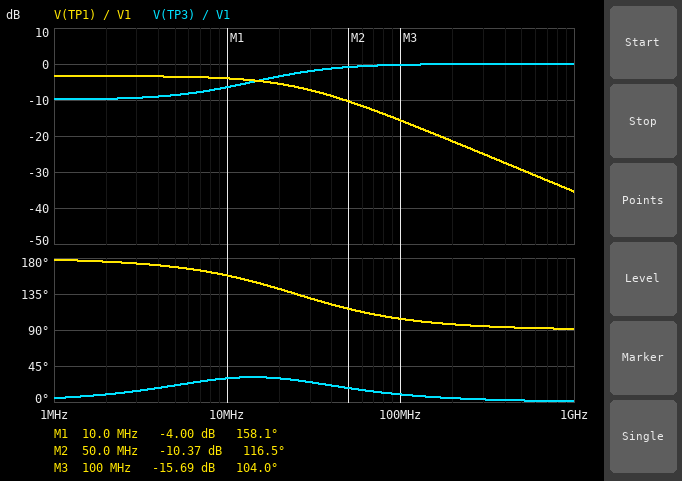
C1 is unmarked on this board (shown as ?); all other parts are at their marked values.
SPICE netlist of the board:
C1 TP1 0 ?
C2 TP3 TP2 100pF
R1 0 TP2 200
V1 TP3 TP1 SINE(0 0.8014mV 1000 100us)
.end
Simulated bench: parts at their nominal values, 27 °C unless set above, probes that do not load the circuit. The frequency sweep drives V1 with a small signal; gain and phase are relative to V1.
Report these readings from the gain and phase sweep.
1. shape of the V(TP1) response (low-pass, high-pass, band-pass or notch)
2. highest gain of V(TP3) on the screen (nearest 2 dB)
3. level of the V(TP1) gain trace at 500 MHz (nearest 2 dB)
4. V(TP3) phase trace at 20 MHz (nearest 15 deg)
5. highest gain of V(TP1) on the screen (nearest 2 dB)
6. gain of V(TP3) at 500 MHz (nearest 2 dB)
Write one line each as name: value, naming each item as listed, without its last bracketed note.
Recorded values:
shape of the V(TP1) response: low-pass
highest gain of V(TP3) on the screen: 0 dB
level of the V(TP1) gain trace at 500 MHz: -30 dB
V(TP3) phase trace at 20 MHz: 30 deg
highest gain of V(TP1) on the screen: -4 dB
gain of V(TP3) at 500 MHz: 0 dB
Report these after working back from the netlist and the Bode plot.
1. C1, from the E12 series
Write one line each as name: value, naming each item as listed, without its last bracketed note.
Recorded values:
C1, from the E12 series: 47 pF
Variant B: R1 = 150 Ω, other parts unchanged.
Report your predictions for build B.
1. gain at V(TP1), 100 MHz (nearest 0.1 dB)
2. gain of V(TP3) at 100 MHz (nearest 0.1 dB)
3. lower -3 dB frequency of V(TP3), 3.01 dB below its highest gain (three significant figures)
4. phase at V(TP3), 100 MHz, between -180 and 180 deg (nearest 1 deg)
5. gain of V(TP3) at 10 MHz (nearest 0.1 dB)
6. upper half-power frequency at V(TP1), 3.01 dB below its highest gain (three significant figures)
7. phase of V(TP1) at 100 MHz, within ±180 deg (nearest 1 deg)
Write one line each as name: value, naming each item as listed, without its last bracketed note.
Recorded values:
gain at V(TP1), 100 MHz: -13.4 dB
gain of V(TP3) at 100 MHz: -0.4 dB
lower -3 dB frequency of V(TP3), 3.01 dB below its highest gain: 29.6 MHz
phase at V(TP3), 100 MHz, between -180 and 180 deg: 12 deg
gain of V(TP3) at 10 MHz: -7.5 dB
upper half-power frequency at V(TP1), 3.01 dB below its highest gain: 33.2 MHz
phase of V(TP1) at 100 MHz, within ±180 deg: 108 deg
